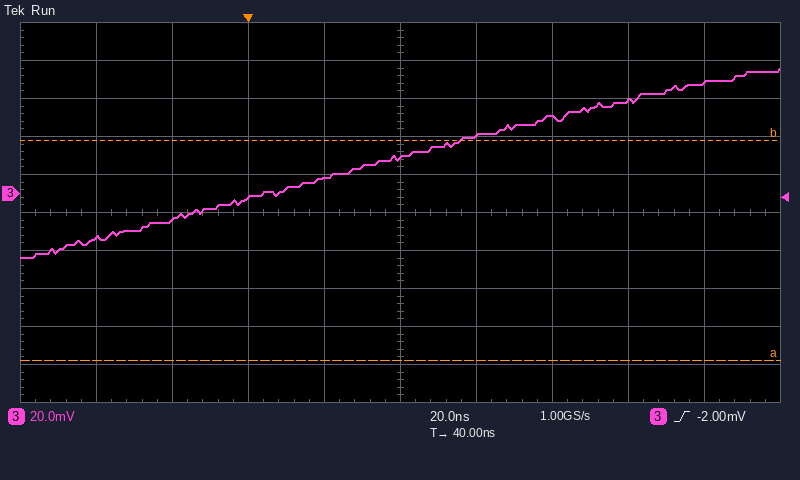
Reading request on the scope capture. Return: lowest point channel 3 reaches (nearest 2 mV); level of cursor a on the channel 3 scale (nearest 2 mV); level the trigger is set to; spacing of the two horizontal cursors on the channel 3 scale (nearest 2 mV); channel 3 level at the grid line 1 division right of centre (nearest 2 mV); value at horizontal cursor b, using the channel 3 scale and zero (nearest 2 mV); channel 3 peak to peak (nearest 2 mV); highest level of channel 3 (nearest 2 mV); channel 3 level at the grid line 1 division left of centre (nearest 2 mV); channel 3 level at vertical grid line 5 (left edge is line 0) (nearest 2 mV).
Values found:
-34 mV
-88 mV
-2.00 mV
116 mV
30 mV
28 mV
100 mV
66 mV
8 mV
18 mV
